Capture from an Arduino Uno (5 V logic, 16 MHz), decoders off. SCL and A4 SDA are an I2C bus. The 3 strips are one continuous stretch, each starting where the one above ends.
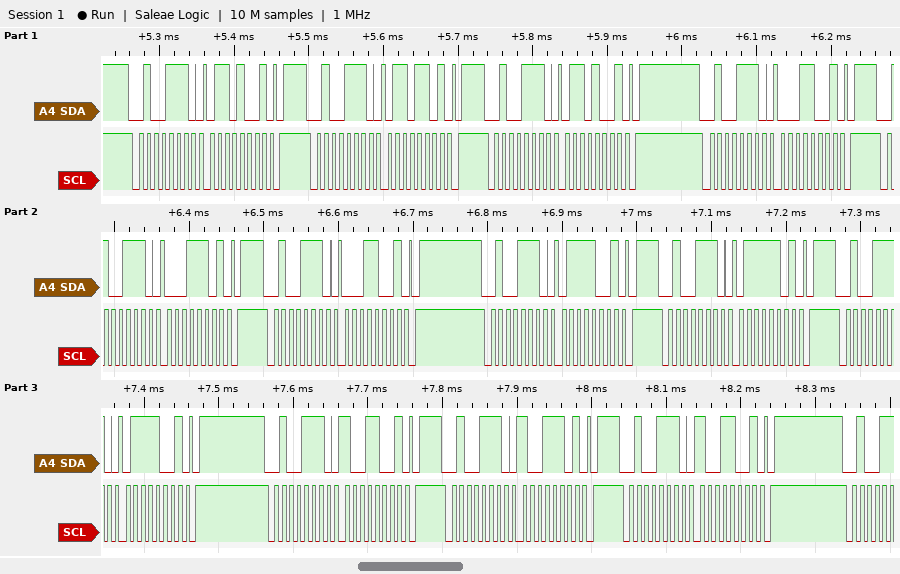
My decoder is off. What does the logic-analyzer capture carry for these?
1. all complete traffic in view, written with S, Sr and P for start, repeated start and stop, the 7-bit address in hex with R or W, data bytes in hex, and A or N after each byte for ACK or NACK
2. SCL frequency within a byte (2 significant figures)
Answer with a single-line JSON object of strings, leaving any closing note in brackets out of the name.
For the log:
{"all complete traffic in view, written with S, Sr and P for start, repeated start and stop, the 7-bit address in hex with R or W, data bytes in hex, and A or N after each byte for ACK or NACK": "S 27W A 69 A P S 27W A 6D A P S 27W A 69 A P S 27W A 19 A P S 27W A 1D A P S 27W A 19 A P S 27W A 79 A P S 27W A 7D A P S 27W A 79 A P S 27W A 99 A P S 27W A 9D A P S 27W A 99 A P", "SCL frequency within a byte": "100 kHz"}
